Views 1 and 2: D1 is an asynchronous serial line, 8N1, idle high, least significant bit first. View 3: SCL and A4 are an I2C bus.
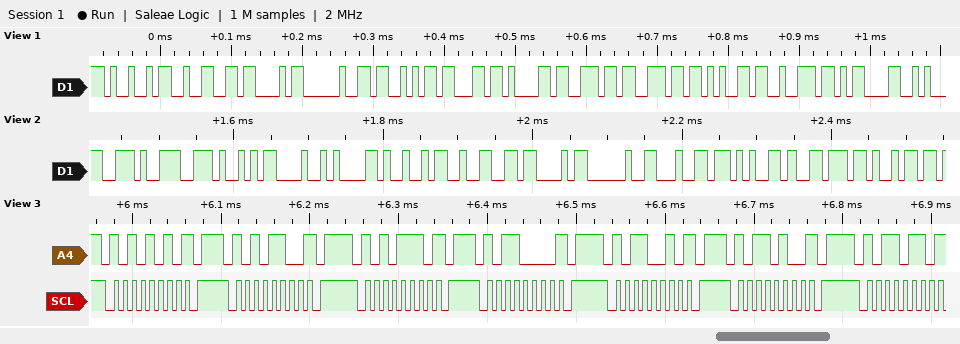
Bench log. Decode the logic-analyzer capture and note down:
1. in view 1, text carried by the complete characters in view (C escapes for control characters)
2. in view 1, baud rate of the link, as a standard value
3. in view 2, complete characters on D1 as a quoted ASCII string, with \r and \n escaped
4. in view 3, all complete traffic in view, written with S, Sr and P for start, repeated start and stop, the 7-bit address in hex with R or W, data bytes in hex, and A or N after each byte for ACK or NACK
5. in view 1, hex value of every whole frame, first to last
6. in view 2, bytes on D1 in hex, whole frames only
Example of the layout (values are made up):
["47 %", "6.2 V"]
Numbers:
["\"I2C Scanner\\r\"", "115200 baud", "\"..\\r\\nI2C devi\"", "S 55W N P S 56W N P S 57W N P S 58W N P S 59W N P S 5AW N P S 5BW N", "49 32 43 20 53 63 61 6E 6E 65 72 0D", "0x2E 0x2E 0x0D 0x0A 0x49 0x32 0x43 0x20 0x64 0x65 0x76 0x69"]
